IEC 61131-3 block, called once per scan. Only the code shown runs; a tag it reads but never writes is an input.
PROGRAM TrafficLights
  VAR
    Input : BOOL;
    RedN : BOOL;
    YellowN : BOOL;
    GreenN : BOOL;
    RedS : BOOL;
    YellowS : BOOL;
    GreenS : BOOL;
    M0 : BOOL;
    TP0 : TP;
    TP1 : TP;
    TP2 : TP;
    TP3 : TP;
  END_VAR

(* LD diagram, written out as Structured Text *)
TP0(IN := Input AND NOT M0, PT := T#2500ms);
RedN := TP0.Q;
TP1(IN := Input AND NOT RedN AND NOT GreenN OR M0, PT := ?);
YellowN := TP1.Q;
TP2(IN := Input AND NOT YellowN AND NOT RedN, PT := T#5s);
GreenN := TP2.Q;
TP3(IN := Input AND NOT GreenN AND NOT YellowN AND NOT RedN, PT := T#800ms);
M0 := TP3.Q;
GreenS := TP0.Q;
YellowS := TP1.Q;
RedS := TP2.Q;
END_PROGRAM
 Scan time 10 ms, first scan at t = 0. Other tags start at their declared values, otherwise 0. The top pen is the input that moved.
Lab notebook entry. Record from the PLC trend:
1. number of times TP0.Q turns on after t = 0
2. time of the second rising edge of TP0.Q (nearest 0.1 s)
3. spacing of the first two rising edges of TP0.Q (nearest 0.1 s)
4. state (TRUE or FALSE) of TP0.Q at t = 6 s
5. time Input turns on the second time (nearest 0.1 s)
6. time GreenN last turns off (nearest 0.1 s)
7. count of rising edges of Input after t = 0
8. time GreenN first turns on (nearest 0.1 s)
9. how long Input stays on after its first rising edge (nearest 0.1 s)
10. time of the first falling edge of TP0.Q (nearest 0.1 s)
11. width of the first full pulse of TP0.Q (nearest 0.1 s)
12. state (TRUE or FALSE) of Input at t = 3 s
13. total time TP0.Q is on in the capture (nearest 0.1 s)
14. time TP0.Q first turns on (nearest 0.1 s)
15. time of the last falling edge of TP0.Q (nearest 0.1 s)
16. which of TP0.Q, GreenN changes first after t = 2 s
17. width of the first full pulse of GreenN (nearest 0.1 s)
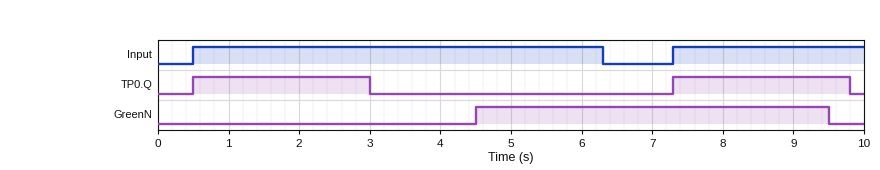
2
7.3 s
6.8 s
FALSE
7.3 s
9.5 s
2
4.5 s
5.8 s
3.0 s
2.5 s
TRUE
5.0 s
0.5 s
9.8 s
TP0.Q
5.0 s
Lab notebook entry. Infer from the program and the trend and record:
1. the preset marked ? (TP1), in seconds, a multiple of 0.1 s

1.5 s
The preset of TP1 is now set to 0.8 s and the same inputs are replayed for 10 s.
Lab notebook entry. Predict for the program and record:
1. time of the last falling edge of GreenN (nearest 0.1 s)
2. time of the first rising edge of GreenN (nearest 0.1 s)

8.8 s
3.8 s
